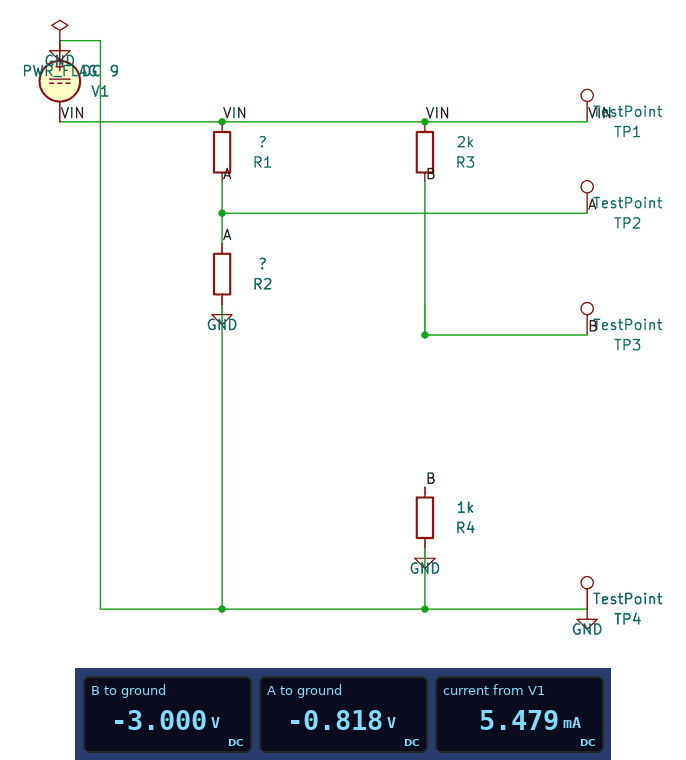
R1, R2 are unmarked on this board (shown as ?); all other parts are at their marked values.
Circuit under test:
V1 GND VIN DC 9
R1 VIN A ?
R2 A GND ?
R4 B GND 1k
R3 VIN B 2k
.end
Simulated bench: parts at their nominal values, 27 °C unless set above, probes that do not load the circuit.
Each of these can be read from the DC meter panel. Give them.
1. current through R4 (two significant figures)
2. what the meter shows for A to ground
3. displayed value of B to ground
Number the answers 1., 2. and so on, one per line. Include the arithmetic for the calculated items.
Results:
1. (0 V - (-3 V)) / 1 kΩ = 3.0 mA
2. -0.818 V
3. -3.000 V
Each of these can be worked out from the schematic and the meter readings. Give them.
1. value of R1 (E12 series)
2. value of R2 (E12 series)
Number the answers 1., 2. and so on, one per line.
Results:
1. 3.3 kΩ
2. 330 Ω
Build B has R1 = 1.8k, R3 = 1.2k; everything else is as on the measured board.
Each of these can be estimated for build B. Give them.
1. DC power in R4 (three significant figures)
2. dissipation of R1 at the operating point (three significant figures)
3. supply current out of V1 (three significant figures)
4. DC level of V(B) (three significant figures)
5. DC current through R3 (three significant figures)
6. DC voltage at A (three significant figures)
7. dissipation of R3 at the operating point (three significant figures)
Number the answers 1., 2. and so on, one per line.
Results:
1. 16.7 mW
2. 32.1 mW
3. 8.32 mA
4. -4.09 V
5. 4.09 mA
6. -1.39 V
7. 20.1 mW
